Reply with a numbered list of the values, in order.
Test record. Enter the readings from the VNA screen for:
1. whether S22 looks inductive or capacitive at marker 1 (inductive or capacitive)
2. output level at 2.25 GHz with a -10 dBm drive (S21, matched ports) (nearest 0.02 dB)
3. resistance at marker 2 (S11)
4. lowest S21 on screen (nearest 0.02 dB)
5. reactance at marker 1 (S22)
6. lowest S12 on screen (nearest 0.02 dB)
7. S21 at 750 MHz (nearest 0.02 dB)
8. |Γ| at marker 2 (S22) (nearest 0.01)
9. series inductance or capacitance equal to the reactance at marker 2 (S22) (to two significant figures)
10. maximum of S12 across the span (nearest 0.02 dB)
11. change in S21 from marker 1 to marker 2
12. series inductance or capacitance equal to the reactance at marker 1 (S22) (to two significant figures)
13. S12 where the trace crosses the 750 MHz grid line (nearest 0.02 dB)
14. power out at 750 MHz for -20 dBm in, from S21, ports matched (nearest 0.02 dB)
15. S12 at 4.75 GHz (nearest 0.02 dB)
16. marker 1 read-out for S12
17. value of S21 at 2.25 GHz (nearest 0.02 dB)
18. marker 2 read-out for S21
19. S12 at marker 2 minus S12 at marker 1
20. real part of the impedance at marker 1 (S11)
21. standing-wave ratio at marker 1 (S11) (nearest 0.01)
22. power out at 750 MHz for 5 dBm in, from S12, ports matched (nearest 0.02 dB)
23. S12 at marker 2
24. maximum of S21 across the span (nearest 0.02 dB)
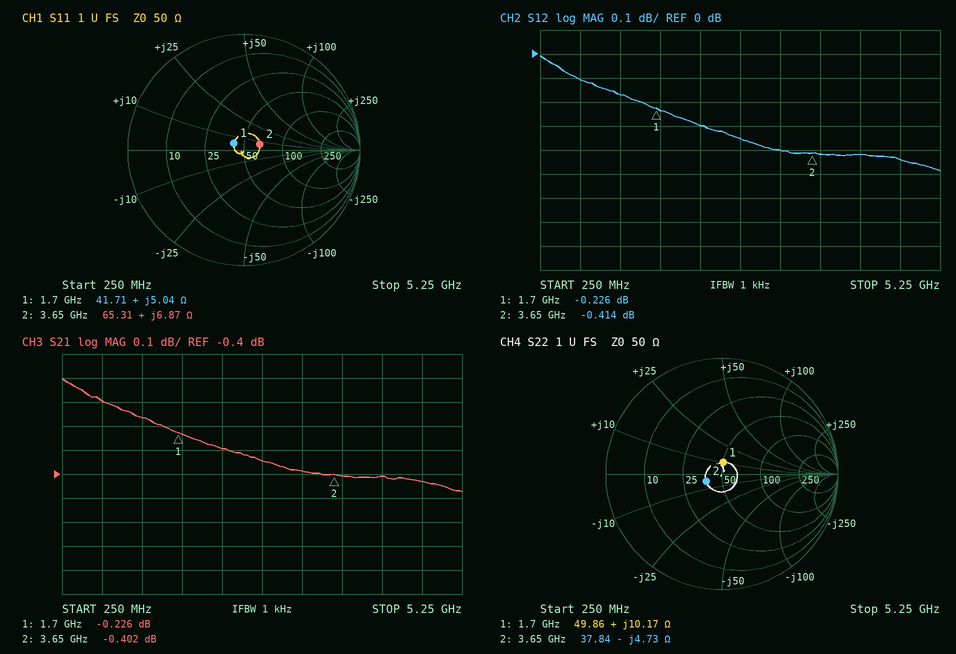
1. inductive
2. -10.30 dBm
3. 65.31 Ω
4. -0.48 dB
5. +10.17 Ω
6. -0.48 dB
7. -0.10 dB
8. 0.15
9. 9.2 pF
10. 0.00 dB
11. -0.176 dB
12. 950 pH
13. -0.10 dB
14. -20.10 dBm
15. -0.44 dB
16. -0.226 dB
17. -0.30 dB
18. -0.402 dB
19. -0.188 dB
20. 41.71 Ω
21. 1.24
22. 4.90 dBm
23. -0.414 dB
24. 0.00 dB
